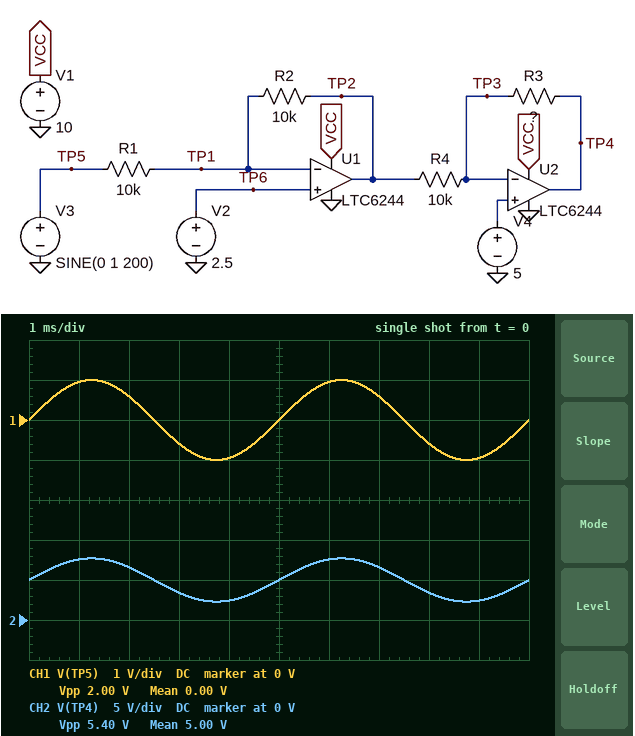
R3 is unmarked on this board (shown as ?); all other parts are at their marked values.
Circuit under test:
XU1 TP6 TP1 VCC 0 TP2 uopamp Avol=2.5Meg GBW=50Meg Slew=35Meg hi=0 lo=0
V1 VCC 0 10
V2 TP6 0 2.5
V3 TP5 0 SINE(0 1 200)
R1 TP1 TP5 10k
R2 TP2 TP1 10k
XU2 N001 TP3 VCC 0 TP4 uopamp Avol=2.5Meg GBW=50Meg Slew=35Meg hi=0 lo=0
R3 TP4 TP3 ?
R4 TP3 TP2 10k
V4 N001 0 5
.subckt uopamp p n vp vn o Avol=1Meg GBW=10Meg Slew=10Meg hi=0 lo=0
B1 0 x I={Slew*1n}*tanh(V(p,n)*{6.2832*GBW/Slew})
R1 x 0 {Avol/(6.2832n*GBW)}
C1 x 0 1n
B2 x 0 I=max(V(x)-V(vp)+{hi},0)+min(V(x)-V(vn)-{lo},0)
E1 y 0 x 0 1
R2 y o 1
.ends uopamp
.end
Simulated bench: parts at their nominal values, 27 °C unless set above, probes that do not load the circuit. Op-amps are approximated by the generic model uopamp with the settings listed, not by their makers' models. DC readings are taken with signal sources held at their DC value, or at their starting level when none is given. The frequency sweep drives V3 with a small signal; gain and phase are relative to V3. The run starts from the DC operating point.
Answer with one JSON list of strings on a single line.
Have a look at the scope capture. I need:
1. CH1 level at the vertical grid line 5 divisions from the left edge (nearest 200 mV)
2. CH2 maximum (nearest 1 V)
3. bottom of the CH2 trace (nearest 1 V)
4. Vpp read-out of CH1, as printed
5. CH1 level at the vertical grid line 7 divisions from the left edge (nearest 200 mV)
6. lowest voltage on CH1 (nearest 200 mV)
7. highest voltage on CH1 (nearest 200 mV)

["0 V", "8 V", "2 V", "2.00 V", "600 mV", "-1.0 V", "1.0 V"]
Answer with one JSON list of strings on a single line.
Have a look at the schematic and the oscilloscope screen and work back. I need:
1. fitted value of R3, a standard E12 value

["27 kΩ"]
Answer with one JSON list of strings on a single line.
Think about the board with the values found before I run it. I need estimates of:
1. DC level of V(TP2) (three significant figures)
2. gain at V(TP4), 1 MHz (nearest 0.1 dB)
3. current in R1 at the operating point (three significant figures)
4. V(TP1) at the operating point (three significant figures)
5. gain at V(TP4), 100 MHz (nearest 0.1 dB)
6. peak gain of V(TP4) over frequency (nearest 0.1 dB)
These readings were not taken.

["5.00 V", "8.6 dB", "250 µA", "2.50 V", "-21.1 dB", "8.6 dB"]
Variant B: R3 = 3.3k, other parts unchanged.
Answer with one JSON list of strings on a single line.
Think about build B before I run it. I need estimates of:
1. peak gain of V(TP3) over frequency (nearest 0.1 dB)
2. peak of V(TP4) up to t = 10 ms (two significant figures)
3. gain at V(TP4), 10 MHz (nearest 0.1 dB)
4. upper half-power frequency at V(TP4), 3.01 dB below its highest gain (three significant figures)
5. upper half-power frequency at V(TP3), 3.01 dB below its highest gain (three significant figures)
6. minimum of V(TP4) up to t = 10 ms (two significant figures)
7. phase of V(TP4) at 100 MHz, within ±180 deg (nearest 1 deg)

["-20.1 dB", "5.3 V", "-10.6 dB", "19.2 MHz", "75.1 MHz", "4.7 V", "-145 deg"]
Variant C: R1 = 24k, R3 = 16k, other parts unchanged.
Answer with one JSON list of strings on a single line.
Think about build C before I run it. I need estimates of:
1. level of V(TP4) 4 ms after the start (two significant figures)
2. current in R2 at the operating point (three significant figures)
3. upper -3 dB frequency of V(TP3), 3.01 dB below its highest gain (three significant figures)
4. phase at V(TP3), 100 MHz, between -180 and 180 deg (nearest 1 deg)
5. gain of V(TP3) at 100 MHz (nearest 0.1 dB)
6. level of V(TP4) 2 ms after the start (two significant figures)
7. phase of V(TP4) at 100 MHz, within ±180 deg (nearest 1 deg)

["6.7 V", "104 µA", "65.0 MHz", "120 deg", "-21.5 dB", "7.7 V", "-150 deg"]
